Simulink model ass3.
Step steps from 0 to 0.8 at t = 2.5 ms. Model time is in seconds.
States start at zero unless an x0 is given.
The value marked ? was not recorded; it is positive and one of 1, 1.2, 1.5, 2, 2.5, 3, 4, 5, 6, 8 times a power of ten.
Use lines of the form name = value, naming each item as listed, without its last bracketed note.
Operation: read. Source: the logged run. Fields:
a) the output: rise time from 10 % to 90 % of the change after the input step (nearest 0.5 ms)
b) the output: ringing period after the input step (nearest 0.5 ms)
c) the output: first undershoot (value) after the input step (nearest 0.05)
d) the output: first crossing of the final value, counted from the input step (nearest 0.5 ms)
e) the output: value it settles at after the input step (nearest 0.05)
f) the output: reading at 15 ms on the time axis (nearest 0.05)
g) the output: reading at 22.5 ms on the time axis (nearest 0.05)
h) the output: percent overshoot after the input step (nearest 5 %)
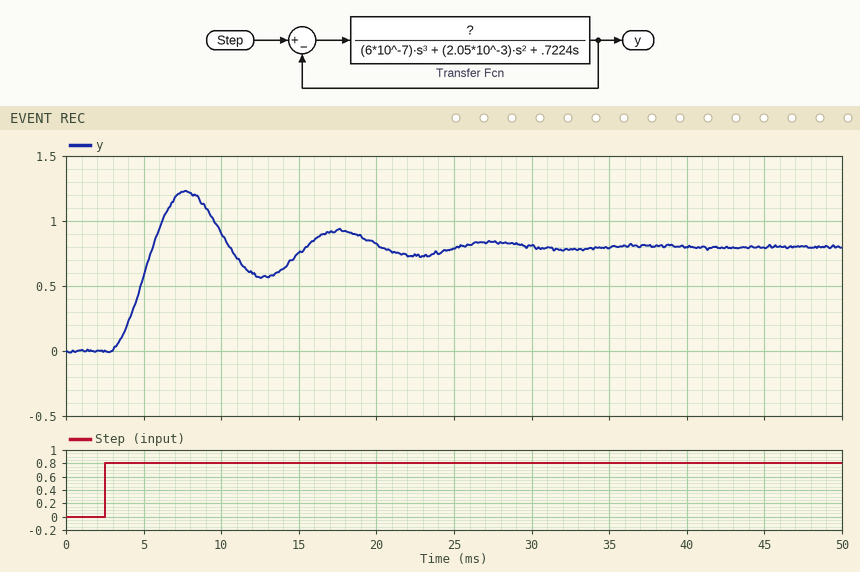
the output: rise time from 10 % to 90 % of the change after the input step = 2.0 ms
the output: ringing period after the input step = 10.0 ms
the output: first undershoot (value) after the input step = 0.55
the output: first crossing of the final value, counted from the input step = 3.0 ms
the output: value it settles at after the input step = 0.80
the output: reading at 15 ms on the time axis = 0.75
the output: reading at 22.5 ms on the time axis = 0.75
the output: percent overshoot after the input step = 55 %
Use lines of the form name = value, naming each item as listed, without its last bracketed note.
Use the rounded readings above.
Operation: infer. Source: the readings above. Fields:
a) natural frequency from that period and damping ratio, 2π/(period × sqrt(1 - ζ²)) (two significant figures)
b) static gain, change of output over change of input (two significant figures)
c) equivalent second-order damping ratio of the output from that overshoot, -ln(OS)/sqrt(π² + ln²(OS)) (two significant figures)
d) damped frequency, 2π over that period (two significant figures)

natural frequency from that period and damping ratio, 2π/(period × sqrt(1 - ζ²)) = 0.64 rad/ms
static gain, change of output over change of input = 1.0
equivalent second-order damping ratio of the output from that overshoot, -ln(OS)/sqrt(π² + ln²(OS)) = 0.19
damped frequency, 2π over that period = 0.63 rad/ms
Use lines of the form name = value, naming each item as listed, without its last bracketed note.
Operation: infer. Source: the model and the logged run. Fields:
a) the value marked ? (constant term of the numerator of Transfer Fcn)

the value marked ? = 800
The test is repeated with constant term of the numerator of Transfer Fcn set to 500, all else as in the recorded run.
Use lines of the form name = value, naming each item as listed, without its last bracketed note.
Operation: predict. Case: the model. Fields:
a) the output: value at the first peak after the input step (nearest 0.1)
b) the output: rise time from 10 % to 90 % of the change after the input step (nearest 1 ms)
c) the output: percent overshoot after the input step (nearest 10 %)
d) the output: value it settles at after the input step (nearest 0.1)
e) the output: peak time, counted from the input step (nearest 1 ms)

the output: value at the first peak after the input step = 1.1
the output: rise time from 10 % to 90 % of the change after the input step = 3 ms
the output: percent overshoot after the input step = 40 %
the output: value it settles at after the input step = 0.8
the output: peak time, counted from the input step = 7 ms
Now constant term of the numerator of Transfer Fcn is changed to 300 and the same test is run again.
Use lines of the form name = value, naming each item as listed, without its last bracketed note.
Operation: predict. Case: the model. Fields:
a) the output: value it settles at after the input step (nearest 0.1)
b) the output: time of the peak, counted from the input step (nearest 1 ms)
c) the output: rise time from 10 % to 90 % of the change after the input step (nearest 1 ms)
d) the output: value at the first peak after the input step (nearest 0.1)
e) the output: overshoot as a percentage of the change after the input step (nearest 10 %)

the output: value it settles at after the input step = 0.8
the output: time of the peak, counted from the input step = 9 ms
the output: rise time from 10 % to 90 % of the change after the input step = 4 ms
the output: value at the first peak after the input step = 1.0
the output: overshoot as a percentage of the change after the input step = 20 %
